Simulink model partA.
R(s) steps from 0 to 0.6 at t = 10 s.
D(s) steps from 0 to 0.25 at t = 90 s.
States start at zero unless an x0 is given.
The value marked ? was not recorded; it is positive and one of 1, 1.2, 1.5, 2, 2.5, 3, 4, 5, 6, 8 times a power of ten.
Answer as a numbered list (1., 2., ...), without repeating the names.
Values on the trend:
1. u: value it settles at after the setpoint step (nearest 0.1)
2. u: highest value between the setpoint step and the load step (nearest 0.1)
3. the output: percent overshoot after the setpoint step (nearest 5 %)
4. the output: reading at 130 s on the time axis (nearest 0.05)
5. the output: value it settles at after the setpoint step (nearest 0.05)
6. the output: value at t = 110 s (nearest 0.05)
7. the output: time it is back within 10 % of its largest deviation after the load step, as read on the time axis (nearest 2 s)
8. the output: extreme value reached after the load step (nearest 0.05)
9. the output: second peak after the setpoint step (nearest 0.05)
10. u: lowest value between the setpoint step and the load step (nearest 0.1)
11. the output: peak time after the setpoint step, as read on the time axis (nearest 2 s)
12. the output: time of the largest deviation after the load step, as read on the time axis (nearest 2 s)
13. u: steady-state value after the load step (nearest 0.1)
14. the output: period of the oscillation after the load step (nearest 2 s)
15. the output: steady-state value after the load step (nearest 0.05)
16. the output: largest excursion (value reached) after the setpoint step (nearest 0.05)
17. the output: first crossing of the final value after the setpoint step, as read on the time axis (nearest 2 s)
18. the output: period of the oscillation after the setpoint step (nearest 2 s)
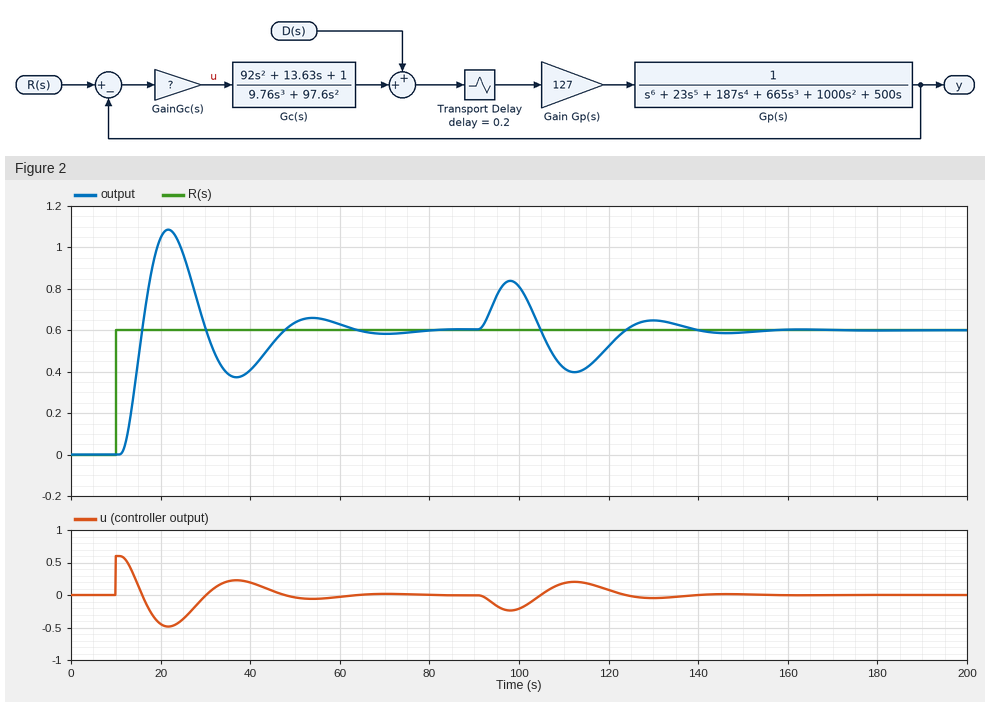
1. 0.0
2. 0.6
3. 80 %
4. 0.65
5. 0.60
6. 0.40
7. 136 s
8. 0.85
9. 0.65
10. -0.5
11. 22 s
12. 98 s
13. 0.0
14. 32 s
15. 0.60
16. 1.10
17. 16 s
18. 32 s
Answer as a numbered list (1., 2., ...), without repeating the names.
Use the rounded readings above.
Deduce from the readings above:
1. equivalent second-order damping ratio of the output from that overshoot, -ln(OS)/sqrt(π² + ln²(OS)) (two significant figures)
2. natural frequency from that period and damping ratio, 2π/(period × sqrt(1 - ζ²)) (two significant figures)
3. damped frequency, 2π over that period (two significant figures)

1. 0.071
2. 0.20 rad/s
3. 0.20 rad/s
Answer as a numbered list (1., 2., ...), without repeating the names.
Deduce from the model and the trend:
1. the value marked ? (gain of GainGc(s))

1. 1
